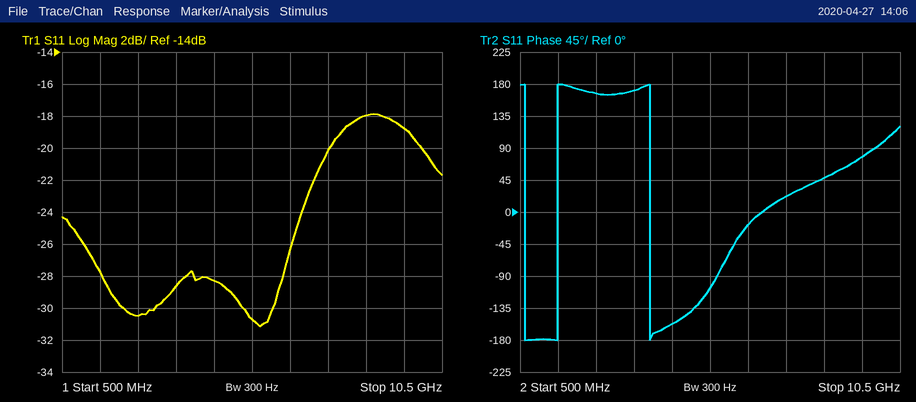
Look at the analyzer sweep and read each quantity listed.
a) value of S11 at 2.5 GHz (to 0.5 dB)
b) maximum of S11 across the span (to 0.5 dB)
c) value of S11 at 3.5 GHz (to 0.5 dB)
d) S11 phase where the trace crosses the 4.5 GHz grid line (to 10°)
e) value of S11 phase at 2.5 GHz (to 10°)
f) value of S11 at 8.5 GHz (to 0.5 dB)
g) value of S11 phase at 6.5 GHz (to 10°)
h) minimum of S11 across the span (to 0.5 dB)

-30.5 dB
-18.0 dB
-28.5 dB
-160°
170°
-18.0 dB
-20°
-31.0 dB
